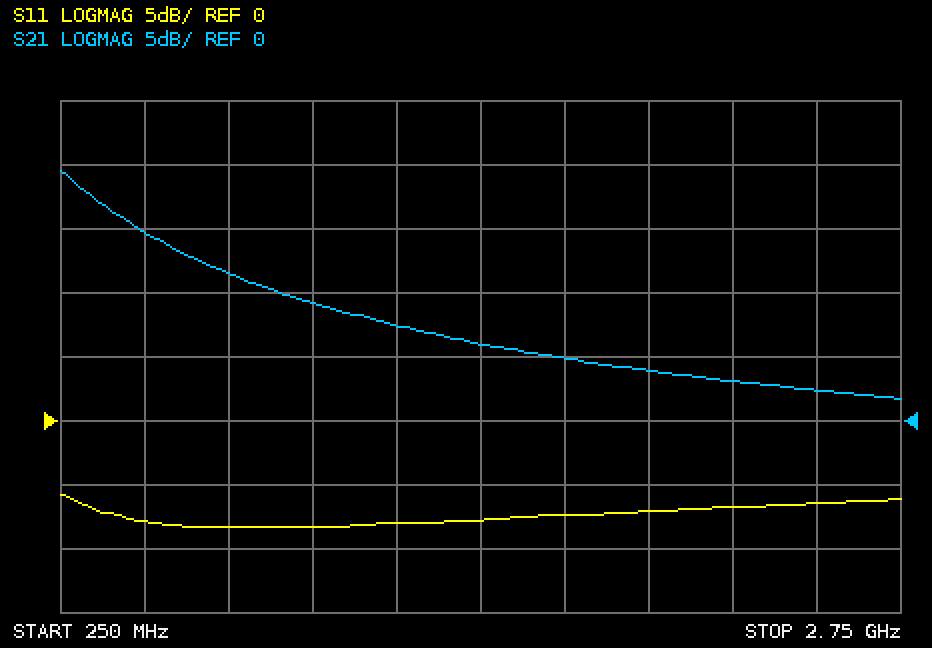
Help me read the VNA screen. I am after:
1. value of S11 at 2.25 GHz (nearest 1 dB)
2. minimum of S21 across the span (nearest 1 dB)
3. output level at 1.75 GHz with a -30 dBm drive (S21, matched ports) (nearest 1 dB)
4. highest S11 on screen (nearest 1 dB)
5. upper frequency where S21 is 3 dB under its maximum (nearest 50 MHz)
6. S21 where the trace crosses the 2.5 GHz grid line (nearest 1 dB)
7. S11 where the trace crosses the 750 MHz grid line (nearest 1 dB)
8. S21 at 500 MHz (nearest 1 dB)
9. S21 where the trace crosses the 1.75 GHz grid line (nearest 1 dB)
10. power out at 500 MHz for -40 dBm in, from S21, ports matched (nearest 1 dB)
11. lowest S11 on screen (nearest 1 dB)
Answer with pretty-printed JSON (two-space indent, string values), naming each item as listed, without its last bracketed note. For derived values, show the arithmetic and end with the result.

{
  "value of S11 at 2.25 GHz": "-7 dB",
  "minimum of S21 across the span": "2 dB",
  "output level at 1.75 GHz with a -30 dBm drive (S21, matched ports)": "-30 dBm + (5 dB) = -25 dBm",
  "highest S11 on screen": "-6 dB",
  "upper frequency where S21 is 3 dB under its maximum": "400 MHz",
  "S21 where the trace crosses the 2.5 GHz grid line": "2 dB",
  "S11 where the trace crosses the 750 MHz grid line": "-8 dB",
  "S21 at 500 MHz": "15 dB",
  "S21 where the trace crosses the 1.75 GHz grid line": "5 dB",
  "power out at 500 MHz for -40 dBm in, from S21, ports matched": "-40 dBm + (15 dB) = -25 dBm",
  "lowest S11 on screen": "-8 dB"
}
